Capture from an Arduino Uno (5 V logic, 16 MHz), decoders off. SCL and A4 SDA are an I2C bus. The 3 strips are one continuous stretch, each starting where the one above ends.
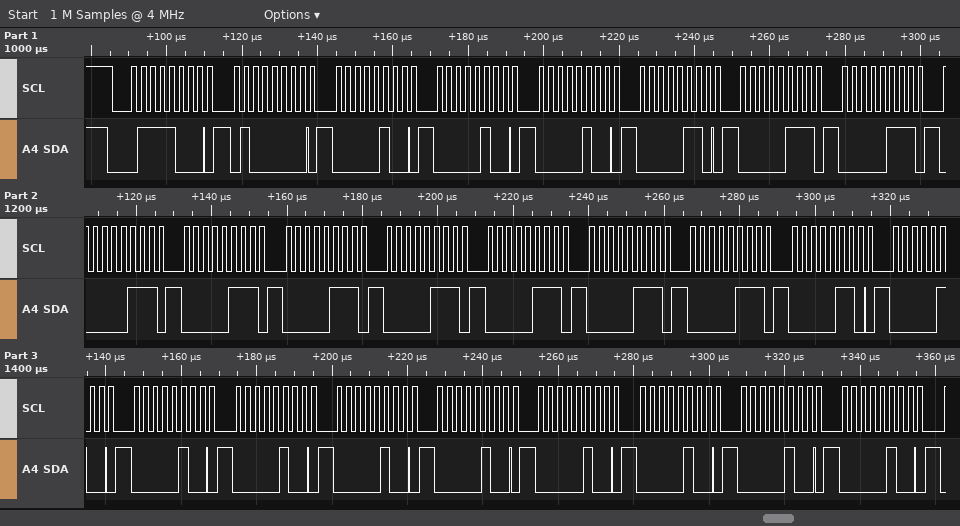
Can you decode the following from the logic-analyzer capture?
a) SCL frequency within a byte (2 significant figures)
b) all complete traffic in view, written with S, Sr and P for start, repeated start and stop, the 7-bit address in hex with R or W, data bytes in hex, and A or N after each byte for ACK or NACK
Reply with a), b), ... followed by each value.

a) 400 kHz
b) S 3CW A 40 A 04 A 04 A 04 A 06 A 07 A 07 A 07 A 07 A 07 A 07 A 07 A 07 A 07 A 06 A 04 A 04 A 04 A 04 A 04 A 04 A 04 A 04 A 04 A
